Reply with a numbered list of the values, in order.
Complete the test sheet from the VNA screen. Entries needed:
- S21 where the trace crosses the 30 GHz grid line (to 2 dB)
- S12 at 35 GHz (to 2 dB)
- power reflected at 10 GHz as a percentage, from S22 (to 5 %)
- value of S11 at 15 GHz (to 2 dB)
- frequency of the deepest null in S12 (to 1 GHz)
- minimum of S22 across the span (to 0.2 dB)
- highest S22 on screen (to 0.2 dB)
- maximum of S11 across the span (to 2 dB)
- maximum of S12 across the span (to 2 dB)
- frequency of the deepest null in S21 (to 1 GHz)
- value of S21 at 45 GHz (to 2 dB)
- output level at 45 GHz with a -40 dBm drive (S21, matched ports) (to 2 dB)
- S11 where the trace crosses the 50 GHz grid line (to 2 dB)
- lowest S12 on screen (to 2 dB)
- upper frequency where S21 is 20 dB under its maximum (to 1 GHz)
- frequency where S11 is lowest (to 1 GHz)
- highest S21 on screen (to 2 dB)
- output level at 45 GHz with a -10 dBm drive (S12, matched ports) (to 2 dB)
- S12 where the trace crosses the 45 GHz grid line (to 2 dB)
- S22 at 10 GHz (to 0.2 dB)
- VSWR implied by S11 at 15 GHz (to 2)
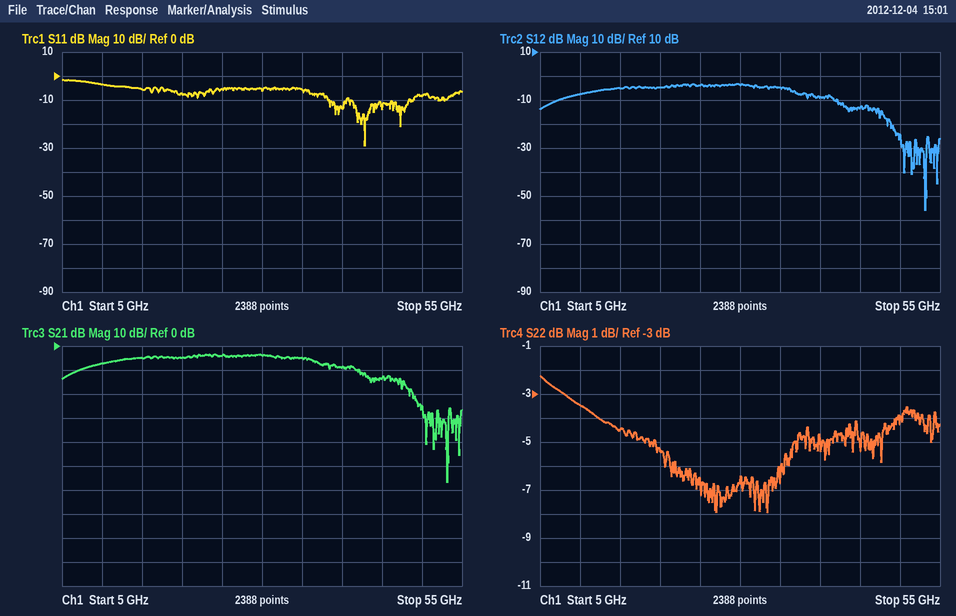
1. -4 dB
2. -4 dB
3. 45 %
4. -6 dB
5. 53 GHz
6. -8.0 dB
7. -2.2 dB
8. -2 dB
9. -4 dB
10. 53 GHz
11. -14 dB
12. -54 dBm
13. -8 dB
14. -56 dB
15. 49 GHz
16. 43 GHz
17. -4 dB
18. -24 dBm
19. -14 dB
20. -3.4 dB
21. 4
